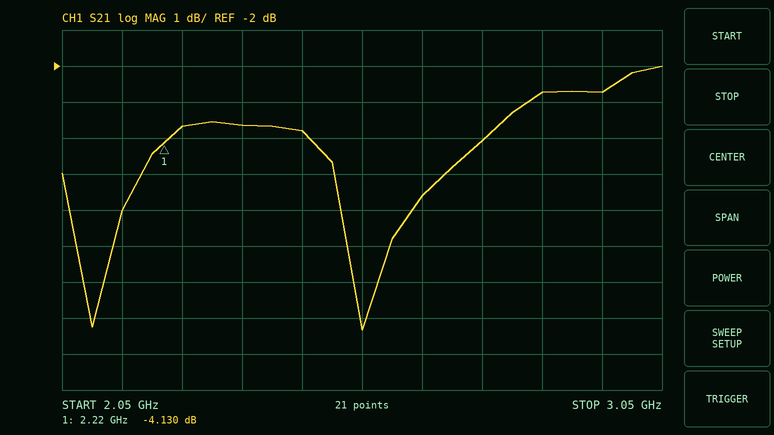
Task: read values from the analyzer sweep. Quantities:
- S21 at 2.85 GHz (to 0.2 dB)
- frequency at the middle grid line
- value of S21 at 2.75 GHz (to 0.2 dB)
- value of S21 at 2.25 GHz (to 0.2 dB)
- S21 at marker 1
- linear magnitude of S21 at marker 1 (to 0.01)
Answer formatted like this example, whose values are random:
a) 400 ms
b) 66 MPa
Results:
a) -2.8 dB
b) 2.55 GHz
c) -4.0 dB
d) -3.6 dB
e) -4.130 dB
f) 0.62
